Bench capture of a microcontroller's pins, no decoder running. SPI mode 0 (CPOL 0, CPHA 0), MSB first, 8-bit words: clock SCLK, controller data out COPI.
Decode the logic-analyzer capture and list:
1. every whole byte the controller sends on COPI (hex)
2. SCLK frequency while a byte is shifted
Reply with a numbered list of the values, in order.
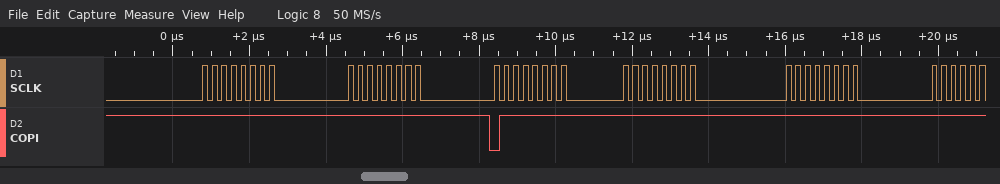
1. FF FF 7F FF FF
2. 4 MHz
